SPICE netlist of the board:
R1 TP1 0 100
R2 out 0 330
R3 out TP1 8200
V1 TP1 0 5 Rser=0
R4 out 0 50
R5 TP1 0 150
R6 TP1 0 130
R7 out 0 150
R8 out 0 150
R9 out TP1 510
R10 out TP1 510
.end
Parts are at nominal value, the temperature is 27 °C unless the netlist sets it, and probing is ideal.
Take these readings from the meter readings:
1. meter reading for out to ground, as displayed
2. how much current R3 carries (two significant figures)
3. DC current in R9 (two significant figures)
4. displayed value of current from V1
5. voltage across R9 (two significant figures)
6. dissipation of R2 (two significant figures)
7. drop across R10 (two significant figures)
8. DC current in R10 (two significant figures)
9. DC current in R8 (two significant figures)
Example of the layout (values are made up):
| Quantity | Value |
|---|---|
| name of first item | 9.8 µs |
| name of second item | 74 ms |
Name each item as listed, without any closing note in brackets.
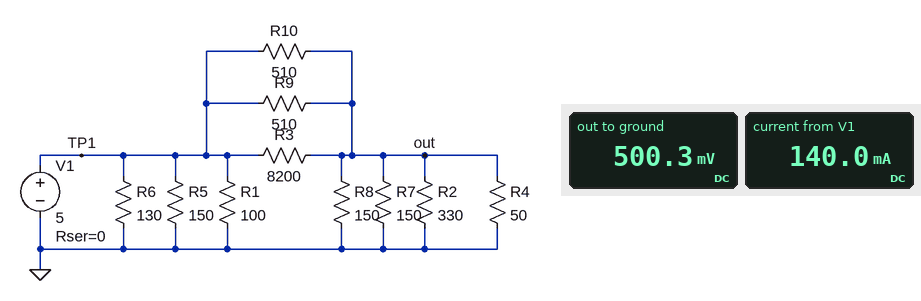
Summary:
| Quantity | Value |
|---|---|
| meter reading for out to ground, as displayed | 500.3 mV |
| how much current R3 carries | 550 µA |
| DC current in R9 | 8.8 mA |
| displayed value of current from V1 | 140.0 mA |
| voltage across R9 | 4.5 V |
| dissipation of R2 | 760 µW |
| drop across R10 | 4.5 V |
| DC current in R10 | 8.8 mA |
| DC current in R8 | 3.3 mA |
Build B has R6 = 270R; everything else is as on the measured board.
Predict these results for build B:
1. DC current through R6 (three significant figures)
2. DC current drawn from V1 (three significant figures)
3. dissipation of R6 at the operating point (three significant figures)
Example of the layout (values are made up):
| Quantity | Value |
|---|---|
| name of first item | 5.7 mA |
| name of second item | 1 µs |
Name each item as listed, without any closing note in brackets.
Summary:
| Quantity | Value |
|---|---|
| DC current through R6 | 18.5 mA |
| DC current drawn from V1 | 120 mA |
| dissipation of R6 at the operating point | 92.6 mW |
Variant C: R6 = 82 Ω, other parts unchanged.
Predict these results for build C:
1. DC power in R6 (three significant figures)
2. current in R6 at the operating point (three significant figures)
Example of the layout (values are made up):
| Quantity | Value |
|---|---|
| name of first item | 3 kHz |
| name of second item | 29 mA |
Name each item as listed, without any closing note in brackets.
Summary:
| Quantity | Value |
|---|---|
| DC power in R6 | 305 mW |
| current in R6 at the operating point | 61.0 mA |
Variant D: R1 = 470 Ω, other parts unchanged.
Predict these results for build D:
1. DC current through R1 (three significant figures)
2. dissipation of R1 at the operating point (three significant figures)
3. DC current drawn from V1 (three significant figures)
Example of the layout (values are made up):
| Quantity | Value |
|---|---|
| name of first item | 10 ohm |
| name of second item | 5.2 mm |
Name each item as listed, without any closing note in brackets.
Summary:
| Quantity | Value |
|---|---|
| DC current through R1 | 10.6 mA |
| dissipation of R1 at the operating point | 53.2 mW |
| DC current drawn from V1 | 101 mA |
